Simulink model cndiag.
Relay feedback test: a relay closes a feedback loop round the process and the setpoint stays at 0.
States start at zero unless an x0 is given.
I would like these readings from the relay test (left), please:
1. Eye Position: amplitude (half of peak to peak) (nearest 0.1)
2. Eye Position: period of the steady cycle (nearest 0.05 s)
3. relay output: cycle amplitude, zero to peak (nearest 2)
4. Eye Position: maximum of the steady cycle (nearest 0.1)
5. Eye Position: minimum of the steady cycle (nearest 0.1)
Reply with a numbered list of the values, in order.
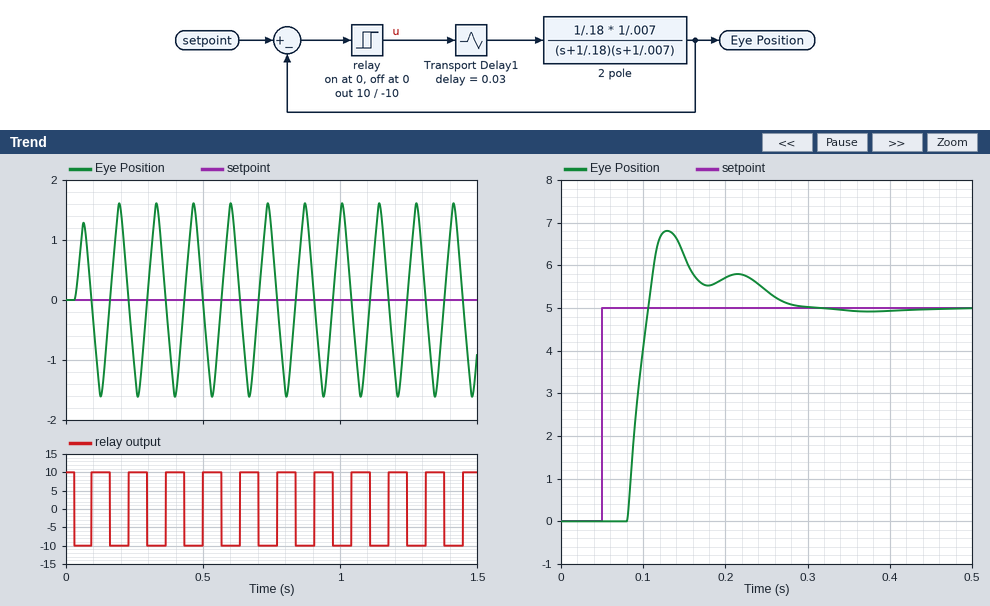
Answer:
1. 1.6
2. 0.15 s
3. 10
4. 1.6
5. -1.6
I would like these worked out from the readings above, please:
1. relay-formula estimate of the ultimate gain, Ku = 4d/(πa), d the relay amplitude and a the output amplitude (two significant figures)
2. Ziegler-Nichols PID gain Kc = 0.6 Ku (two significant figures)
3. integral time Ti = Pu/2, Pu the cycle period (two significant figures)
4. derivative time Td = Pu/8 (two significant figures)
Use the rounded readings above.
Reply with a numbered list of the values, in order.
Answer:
1. 8.0
2. 4.8
3. 0.075 s
4. 0.019 s
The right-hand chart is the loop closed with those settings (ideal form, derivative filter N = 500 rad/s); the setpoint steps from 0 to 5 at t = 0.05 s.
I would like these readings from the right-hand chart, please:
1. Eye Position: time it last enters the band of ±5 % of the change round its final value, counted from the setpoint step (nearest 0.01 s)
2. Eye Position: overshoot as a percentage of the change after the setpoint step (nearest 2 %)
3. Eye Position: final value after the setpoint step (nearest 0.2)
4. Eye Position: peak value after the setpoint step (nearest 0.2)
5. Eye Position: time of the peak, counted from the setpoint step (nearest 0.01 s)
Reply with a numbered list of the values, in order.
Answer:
1. 0.21 s
2. 36 %
3. 5.0
4. 6.8
5. 0.08 s
